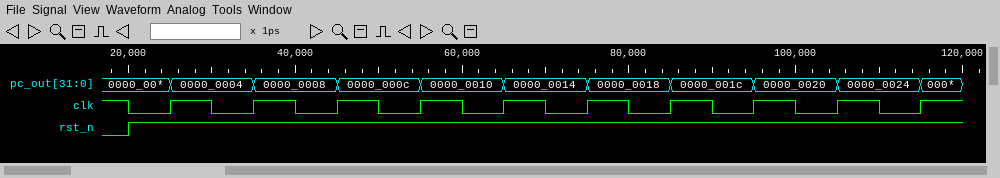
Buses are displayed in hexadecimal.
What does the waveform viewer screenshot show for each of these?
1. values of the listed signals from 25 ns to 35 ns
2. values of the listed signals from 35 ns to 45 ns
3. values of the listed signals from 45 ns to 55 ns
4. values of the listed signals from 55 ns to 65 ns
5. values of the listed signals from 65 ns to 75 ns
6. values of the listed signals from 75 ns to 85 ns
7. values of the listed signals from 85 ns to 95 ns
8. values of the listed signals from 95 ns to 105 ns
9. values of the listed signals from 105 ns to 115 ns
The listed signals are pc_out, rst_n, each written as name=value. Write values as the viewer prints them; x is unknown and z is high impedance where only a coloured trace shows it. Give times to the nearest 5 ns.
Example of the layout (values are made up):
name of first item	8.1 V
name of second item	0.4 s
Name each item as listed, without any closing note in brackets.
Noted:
values of the listed signals from 25 ns to 35 ns	pc_out=0000_0004, rst_n=1
values of the listed signals from 35 ns to 45 ns	pc_out=0000_0008, rst_n=1
values of the listed signals from 45 ns to 55 ns	pc_out=0000_000c, rst_n=1
values of the listed signals from 55 ns to 65 ns	pc_out=0000_0010, rst_n=1
values of the listed signals from 65 ns to 75 ns	pc_out=0000_0014, rst_n=1
values of the listed signals from 75 ns to 85 ns	pc_out=0000_0018, rst_n=1
values of the listed signals from 85 ns to 95 ns	pc_out=0000_001c, rst_n=1
values of the listed signals from 95 ns to 105 ns	pc_out=0000_0020, rst_n=1
values of the listed signals from 105 ns to 115 ns	pc_out=0000_0024, rst_n=1
